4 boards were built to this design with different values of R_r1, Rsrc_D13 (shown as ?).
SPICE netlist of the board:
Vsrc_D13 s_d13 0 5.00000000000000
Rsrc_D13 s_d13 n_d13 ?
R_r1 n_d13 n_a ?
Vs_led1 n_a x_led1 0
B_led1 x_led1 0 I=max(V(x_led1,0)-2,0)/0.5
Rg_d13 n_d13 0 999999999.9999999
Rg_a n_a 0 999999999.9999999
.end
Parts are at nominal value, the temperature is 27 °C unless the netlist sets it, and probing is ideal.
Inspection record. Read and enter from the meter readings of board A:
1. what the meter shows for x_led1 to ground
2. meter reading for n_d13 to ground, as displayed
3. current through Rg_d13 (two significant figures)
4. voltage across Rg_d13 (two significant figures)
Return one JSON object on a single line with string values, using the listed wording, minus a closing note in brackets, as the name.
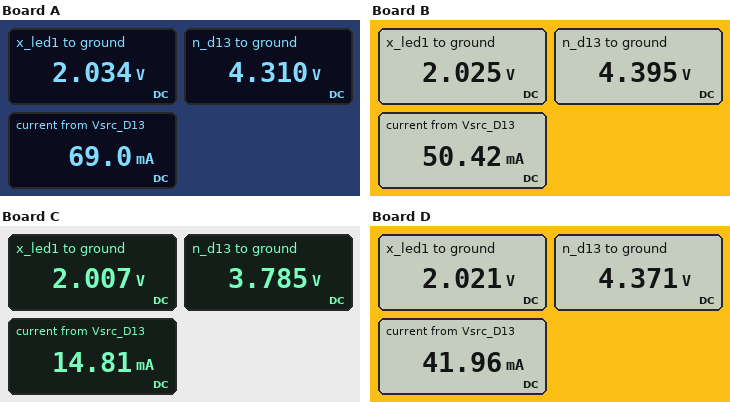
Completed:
{"what the meter shows for x_led1 to ground": "2.034 V", "meter reading for n_d13 to ground, as displayed": "4.310 V", "current through Rg_d13": "4.3 nA", "voltage across Rg_d13": "4.3 V"}
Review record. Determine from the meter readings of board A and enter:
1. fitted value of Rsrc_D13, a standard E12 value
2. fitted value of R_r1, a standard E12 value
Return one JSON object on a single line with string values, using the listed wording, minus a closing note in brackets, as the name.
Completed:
{"fitted value of Rsrc_D13, a standard E12 value": "10 Ω", "fitted value of R_r1, a standard E12 value": "33 Ω"}
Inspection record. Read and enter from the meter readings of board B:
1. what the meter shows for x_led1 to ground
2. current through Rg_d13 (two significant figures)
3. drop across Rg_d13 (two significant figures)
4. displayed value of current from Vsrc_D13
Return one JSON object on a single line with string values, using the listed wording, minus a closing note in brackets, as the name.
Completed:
{"what the meter shows for x_led1 to ground": "2.025 V", "current through Rg_d13": "4.4 nA", "drop across Rg_d13": "4.4 V", "displayed value of current from Vsrc_D13": "50.42 mA"}
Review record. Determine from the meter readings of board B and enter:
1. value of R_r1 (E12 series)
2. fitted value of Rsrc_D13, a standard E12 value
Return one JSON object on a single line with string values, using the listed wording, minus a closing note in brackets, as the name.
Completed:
{"value of R_r1": "47 Ω", "fitted value of Rsrc_D13, a standard E12 value": "12 Ω"}
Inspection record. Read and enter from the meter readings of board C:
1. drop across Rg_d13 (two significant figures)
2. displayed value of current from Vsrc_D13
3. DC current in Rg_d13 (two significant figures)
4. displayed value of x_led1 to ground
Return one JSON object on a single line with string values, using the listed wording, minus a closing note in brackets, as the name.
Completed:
{"drop across Rg_d13": "3.8 V", "displayed value of current from Vsrc_D13": "14.81 mA", "DC current in Rg_d13": "3.8 nA", "displayed value of x_led1 to ground": "2.007 V"}
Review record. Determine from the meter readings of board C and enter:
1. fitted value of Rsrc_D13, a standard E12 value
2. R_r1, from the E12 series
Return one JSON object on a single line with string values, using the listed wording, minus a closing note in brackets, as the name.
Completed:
{"fitted value of Rsrc_D13, a standard E12 value": "82 Ω", "R_r1, from the E12 series": "120 Ω"}
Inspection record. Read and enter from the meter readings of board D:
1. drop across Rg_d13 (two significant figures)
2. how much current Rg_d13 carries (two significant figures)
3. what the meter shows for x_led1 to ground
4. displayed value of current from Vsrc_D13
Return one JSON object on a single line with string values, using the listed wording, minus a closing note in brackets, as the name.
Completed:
{"drop across Rg_d13": "4.4 V", "how much current Rg_d13 carries": "4.4 nA", "what the meter shows for x_led1 to ground": "2.021 V", "displayed value of current from Vsrc_D13": "41.96 mA"}
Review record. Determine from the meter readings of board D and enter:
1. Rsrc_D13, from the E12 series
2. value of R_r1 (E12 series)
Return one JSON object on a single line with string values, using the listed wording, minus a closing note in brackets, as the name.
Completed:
{"Rsrc_D13, from the E12 series": "15 Ω", "value of R_r1": "56 Ω"}
